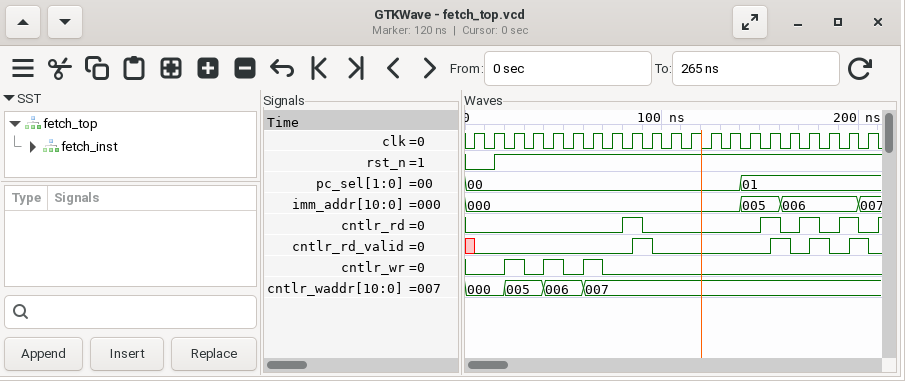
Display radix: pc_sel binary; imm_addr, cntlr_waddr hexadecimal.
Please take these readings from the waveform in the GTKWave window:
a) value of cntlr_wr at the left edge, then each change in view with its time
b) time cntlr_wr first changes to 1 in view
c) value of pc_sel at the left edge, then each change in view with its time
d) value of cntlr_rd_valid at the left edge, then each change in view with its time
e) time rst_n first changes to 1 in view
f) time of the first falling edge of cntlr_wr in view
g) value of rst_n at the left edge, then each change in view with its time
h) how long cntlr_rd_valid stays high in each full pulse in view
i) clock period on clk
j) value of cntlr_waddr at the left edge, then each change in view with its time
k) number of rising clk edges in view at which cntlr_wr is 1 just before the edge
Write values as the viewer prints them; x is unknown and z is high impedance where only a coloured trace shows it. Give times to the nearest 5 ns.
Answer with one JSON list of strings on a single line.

["0, 1 at 20 ns, 0 at 30 ns, 1 at 40 ns, 0 at 50 ns, 1 at 60 ns, 0 at 70 ns", "20 ns", "00, 01 at 140 ns", "x, 0 at 5 ns, 1 at 85 ns, 0 at 95 ns, 1 at 155 ns, 0 at 165 ns, 1 at 175 ns, 0 at 185 ns, 1 at 195 ns, 0 at 205 ns", "15 ns", "30 ns", "0, 1 at 15 ns", "10 ns, 10 ns, 10 ns, 10 ns", "10 ns", "000, 005 at 20 ns, 006 at 40 ns, 007 at 60 ns", "3"]
